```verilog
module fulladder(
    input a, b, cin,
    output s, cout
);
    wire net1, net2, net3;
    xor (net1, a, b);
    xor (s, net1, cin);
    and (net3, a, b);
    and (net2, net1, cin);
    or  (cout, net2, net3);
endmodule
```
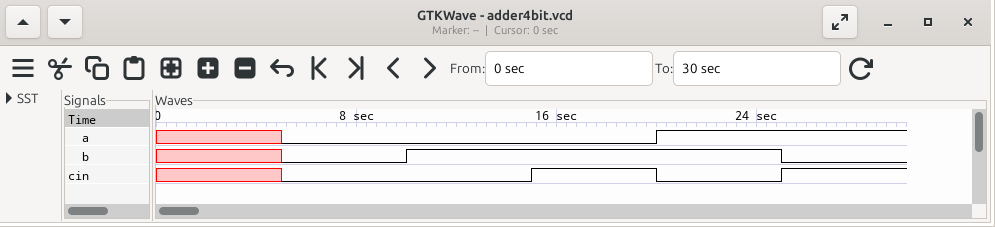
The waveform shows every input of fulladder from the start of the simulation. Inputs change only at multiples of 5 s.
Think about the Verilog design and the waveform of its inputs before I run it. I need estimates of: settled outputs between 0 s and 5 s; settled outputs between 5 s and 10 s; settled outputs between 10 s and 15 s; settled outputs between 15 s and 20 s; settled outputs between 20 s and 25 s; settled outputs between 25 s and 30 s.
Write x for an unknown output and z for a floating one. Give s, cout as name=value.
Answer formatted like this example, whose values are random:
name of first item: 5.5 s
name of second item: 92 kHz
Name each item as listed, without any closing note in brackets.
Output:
settled outputs between 0 s and 5 s: s=x, cout=x
settled outputs between 5 s and 10 s: s=0, cout=0
settled outputs between 10 s and 15 s: s=1, cout=0
settled outputs between 15 s and 20 s: s=0, cout=1
settled outputs between 20 s and 25 s: s=0, cout=1
settled outputs between 25 s and 30 s: s=0, cout=1
